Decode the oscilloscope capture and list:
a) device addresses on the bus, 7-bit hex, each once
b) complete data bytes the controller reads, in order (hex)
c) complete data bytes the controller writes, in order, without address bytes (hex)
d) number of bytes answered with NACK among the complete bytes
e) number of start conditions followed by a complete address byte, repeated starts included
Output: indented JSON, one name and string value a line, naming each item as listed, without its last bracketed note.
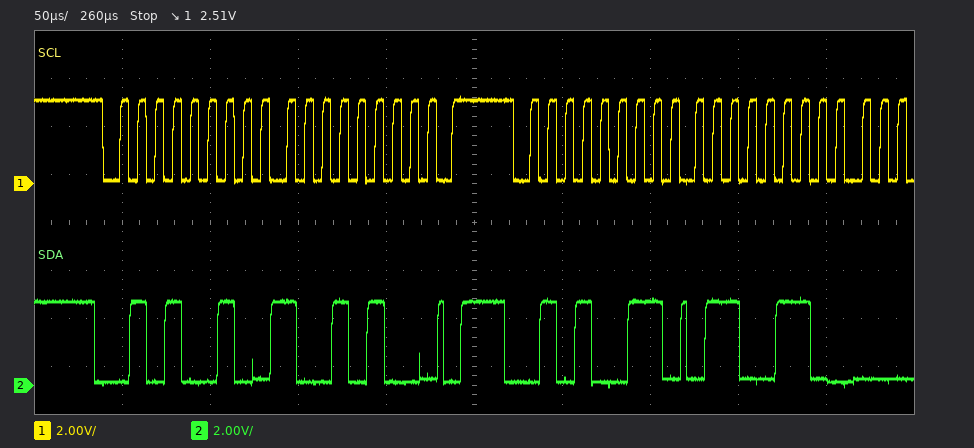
{
  "device addresses on the bus, 7-bit hex, each once": "0x29",
  "complete data bytes the controller reads, in order": "66",
  "complete data bytes the controller writes, in order, without address bytes": "94",
  "number of bytes answered with NACK among the complete bytes": "0",
  "number of start conditions followed by a complete address byte, repeated starts included": "2"
}
